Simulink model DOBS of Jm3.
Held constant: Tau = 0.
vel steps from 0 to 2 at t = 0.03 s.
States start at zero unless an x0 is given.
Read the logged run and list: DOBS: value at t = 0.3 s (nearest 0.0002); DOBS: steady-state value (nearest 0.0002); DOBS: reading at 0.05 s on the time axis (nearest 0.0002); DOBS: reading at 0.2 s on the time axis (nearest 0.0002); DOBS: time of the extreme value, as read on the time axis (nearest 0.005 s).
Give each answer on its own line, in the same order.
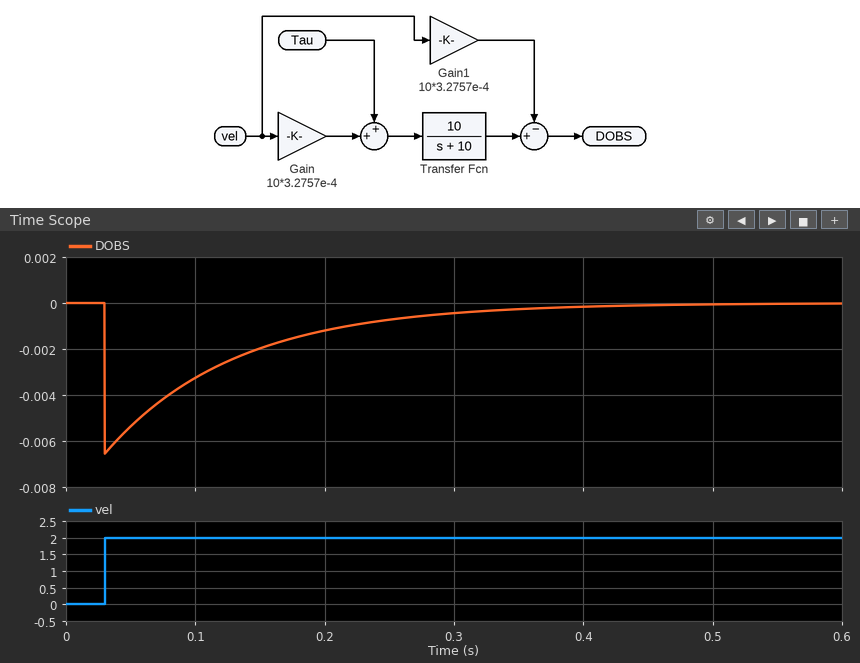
-0.0004
0.0000
-0.0054
-0.0012
0.030 s
